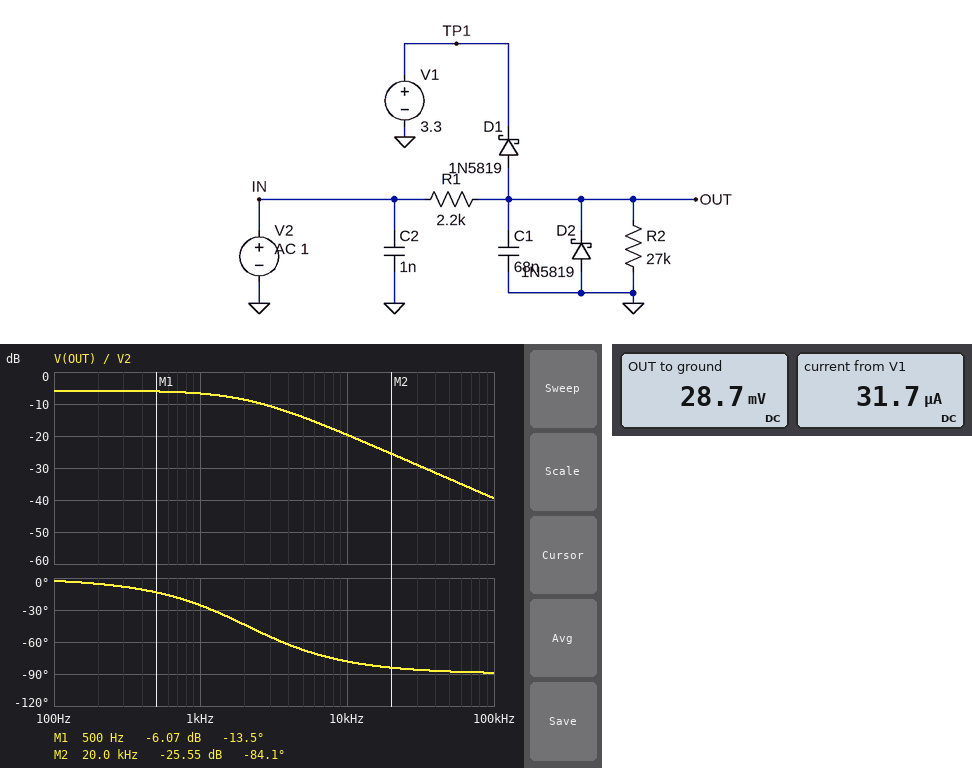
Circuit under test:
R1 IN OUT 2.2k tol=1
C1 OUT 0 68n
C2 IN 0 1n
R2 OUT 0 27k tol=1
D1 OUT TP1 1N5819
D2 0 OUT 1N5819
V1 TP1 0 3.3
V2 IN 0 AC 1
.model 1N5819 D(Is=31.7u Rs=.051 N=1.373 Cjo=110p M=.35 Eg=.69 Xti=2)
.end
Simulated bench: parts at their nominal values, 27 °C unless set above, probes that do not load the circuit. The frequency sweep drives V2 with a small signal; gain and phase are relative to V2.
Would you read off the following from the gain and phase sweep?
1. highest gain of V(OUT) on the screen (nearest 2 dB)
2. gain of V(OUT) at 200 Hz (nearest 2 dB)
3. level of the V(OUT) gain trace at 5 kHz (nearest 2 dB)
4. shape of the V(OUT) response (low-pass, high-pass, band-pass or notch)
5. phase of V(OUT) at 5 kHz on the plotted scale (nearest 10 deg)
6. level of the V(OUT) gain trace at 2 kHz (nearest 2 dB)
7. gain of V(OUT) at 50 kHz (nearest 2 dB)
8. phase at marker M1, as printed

-6 dB
-6 dB
-14 dB
low-pass
-70 deg
-8 dB
-34 dB
-13.5 deg
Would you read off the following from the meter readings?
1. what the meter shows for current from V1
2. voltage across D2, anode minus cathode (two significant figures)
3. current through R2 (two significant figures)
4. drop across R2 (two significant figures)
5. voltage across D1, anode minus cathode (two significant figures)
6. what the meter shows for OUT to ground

31.7 µA
-29 mV
1.1 µA
29 mV
-3.3 V
28.7 mV
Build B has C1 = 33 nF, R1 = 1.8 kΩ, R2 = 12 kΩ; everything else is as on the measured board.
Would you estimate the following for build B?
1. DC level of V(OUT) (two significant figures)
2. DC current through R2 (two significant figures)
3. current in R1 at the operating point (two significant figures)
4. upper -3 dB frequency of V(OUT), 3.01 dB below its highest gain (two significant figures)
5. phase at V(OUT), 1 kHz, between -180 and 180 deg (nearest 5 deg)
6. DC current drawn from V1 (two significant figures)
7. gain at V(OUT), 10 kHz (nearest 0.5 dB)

25 mV
2.1 µA
14 µA
5.2 kHz
-10 deg
32 µA
-12.5 dB
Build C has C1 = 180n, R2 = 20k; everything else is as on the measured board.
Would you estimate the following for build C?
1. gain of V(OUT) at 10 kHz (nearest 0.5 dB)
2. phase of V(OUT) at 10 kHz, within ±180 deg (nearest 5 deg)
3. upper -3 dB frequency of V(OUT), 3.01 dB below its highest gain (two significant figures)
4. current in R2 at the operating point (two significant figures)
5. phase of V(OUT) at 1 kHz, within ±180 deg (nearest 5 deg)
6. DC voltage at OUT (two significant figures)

-28.0 dB
-85 deg
800 Hz
1.4 µA
-50 deg
28 mV
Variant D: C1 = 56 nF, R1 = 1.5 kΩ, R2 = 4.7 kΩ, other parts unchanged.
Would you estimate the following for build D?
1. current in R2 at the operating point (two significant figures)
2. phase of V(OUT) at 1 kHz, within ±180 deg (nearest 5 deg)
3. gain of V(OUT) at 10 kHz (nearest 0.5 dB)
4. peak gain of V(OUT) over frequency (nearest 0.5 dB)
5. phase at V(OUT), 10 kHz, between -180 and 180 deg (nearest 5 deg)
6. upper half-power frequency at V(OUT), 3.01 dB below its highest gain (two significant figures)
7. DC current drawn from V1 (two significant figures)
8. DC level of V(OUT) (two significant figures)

4.3 µA
-15 deg
-15.0 dB
-6.5 dB
-70 deg
3.9 kHz
32 µA
20 mV
